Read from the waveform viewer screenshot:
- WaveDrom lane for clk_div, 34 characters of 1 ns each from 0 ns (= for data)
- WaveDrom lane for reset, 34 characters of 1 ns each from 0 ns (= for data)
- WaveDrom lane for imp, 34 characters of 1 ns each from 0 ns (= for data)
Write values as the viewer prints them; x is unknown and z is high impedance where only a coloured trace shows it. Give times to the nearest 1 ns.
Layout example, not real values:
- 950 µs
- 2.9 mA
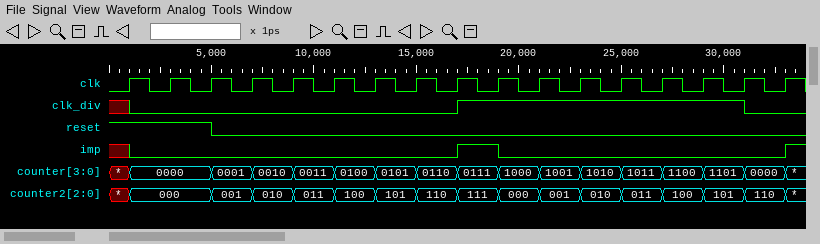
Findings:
- {name: 'clk_div', wave: 'x0...............1.............0..'}
- {name: 'reset', wave: '1....0............................'}
- {name: 'imp', wave: 'x0...............1.0.............1'}
